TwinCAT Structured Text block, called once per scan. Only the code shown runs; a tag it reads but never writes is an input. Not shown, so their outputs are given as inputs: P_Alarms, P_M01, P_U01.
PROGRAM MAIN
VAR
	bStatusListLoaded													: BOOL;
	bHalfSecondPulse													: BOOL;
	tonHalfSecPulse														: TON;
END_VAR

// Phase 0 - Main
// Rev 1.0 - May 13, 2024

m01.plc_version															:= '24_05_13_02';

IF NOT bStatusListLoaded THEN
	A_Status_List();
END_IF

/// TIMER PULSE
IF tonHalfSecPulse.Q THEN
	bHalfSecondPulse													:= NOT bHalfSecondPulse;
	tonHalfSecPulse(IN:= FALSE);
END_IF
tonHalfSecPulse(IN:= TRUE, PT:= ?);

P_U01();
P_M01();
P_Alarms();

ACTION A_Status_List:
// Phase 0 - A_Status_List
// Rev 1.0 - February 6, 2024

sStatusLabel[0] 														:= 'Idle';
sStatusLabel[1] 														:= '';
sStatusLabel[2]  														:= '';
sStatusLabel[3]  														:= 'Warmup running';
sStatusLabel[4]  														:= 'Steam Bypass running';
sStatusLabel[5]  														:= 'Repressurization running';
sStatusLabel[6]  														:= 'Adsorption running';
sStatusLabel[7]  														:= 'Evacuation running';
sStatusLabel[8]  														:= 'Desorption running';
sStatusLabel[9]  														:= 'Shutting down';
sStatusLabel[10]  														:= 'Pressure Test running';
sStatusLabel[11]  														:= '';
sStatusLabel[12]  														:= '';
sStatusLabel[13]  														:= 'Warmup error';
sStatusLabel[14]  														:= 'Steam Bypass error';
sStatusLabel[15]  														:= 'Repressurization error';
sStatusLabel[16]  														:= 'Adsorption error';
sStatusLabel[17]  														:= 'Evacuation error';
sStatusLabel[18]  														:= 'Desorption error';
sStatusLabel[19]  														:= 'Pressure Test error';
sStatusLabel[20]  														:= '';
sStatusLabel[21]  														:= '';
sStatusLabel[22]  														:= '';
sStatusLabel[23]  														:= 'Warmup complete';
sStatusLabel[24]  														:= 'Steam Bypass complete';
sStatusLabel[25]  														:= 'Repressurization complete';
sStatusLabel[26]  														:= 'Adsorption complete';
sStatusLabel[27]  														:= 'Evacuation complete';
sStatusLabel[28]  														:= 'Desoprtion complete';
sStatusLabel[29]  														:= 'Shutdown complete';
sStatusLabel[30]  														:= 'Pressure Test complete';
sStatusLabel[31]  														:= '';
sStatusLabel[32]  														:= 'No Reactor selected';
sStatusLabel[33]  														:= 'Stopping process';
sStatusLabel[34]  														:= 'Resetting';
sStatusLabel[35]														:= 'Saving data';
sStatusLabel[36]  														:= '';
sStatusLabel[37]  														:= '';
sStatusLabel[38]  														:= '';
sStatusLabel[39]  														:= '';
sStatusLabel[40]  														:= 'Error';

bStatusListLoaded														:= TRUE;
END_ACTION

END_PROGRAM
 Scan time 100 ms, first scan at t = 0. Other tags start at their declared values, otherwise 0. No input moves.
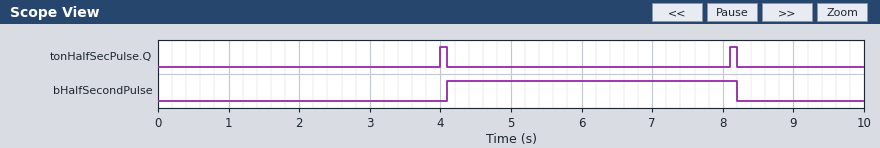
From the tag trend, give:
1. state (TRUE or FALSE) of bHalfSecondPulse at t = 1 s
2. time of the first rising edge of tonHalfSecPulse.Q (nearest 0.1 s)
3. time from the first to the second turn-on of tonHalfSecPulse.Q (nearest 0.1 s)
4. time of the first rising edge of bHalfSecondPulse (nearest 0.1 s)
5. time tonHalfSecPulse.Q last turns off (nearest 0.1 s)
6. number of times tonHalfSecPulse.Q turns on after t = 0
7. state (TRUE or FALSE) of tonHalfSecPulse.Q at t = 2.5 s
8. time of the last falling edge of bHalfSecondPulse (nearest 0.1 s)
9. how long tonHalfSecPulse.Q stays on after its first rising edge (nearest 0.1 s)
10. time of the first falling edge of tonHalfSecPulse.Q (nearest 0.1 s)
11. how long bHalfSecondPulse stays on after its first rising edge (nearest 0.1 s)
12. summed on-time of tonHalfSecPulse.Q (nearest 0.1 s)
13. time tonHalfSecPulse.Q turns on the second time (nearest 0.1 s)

FALSE
4.0 s
4.1 s
4.1 s
8.2 s
2
FALSE
8.2 s
0.1 s
4.1 s
4.1 s
0.2 s
8.1 s
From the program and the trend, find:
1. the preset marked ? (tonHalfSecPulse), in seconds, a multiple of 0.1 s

4.0 s
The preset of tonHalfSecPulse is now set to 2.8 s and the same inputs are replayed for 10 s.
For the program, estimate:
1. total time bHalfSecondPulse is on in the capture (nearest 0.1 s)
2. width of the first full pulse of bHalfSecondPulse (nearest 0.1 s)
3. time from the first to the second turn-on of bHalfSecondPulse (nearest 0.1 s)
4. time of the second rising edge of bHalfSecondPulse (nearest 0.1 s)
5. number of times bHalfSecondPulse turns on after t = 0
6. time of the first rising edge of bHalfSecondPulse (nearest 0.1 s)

4.2 s
2.9 s
5.8 s
8.7 s
2
2.9 s
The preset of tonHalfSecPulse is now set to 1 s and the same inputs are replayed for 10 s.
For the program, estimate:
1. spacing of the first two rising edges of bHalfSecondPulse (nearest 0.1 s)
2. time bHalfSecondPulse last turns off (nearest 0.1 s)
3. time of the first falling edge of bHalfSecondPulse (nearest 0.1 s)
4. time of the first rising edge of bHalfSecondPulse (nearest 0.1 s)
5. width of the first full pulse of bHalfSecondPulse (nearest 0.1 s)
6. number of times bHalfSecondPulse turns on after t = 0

2.2 s
8.8 s
2.2 s
1.1 s
1.1 s
5
